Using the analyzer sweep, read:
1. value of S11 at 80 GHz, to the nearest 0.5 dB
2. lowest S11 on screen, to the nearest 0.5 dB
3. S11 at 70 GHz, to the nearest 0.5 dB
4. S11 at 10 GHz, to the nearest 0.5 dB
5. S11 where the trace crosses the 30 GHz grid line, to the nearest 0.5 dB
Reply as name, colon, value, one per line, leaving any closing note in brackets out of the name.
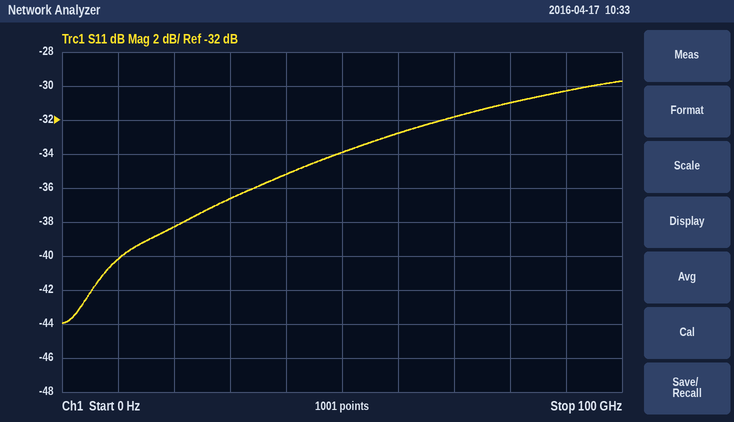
value of S11 at 80 GHz, to the nearest 0.5 dB: -31.0 dB
lowest S11 on screen, to the nearest 0.5 dB: -44.0 dB
S11 at 70 GHz, to the nearest 0.5 dB: -32.0 dB
S11 at 10 GHz, to the nearest 0.5 dB: -40.0 dB
S11 where the trace crosses the 30 GHz grid line, to the nearest 0.5 dB: -36.5 dB
